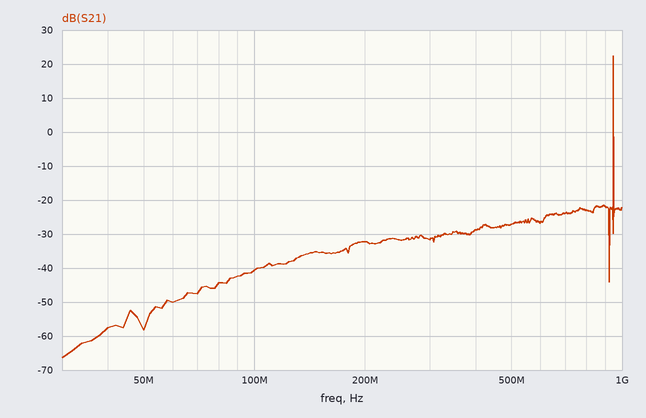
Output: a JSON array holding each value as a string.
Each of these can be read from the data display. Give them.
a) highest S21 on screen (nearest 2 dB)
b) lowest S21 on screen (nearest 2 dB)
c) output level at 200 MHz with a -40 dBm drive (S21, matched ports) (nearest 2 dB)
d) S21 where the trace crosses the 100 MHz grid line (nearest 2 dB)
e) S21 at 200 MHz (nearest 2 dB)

["22 dB", "-66 dB", "-72 dBm", "-40 dB", "-32 dB"]
